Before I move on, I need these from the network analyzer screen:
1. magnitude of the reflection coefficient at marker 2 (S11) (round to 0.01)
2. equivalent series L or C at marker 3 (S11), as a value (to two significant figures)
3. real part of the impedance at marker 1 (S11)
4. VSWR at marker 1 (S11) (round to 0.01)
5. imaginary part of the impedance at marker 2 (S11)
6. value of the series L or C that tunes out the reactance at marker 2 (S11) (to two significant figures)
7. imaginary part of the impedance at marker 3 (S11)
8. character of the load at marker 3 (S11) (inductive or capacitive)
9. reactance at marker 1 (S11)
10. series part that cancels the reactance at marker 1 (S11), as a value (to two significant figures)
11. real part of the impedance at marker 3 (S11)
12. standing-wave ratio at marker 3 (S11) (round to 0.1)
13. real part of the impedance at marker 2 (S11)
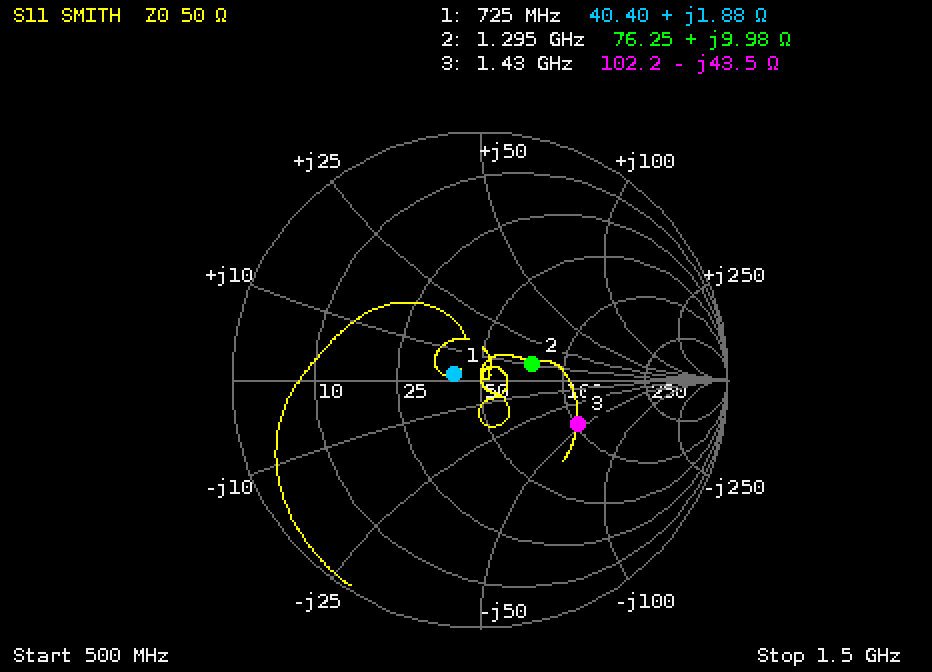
0.22
2.6 pF
40.40 Ω
1.24
+9.98 Ω
12 pF
-43.5 Ω
capacitive
+1.88 Ω
120 pF
102.2 Ω
2.5
76.25 Ω
